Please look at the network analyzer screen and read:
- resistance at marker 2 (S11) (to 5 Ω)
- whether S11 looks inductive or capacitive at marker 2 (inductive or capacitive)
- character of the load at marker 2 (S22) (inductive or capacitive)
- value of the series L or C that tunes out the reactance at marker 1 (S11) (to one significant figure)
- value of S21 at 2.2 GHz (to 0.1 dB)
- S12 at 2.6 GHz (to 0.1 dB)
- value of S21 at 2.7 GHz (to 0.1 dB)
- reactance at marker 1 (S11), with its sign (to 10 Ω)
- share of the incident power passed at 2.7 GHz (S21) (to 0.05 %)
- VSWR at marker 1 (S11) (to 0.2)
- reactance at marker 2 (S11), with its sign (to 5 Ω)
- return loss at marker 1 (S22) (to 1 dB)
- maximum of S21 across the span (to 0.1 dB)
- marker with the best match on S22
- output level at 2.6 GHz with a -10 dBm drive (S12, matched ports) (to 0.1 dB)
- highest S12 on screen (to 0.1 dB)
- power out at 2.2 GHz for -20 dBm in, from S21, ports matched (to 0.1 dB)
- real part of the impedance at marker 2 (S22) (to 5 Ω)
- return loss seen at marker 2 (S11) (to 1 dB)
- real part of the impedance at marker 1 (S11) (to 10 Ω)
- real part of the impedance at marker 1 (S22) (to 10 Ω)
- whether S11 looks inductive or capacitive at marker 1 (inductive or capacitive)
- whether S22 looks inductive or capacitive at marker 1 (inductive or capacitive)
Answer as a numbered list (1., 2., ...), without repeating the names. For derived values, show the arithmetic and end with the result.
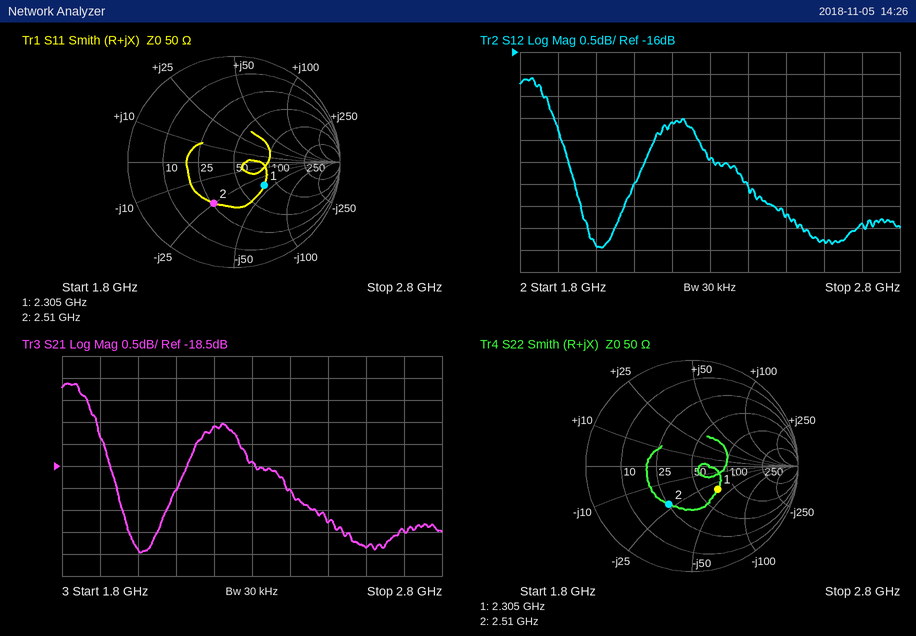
1. 25 Ω
2. capacitive
3. capacitive
4. L = 40 Ω/(2π × 2.305 GHz) ≈ 3 nH
5. -17.6 dB
6. -20.3 dB
7. -20.0 dB
8. -40 Ω
9. 10^(-20/10) ≈ 1.00 %
10. 2.2
11. -25 Ω
12. 10 dB
13. -16.6 dB
14. marker 1
15. -10 dBm + (-20.3 dB) = -30.3 dBm
16. -16.6 dB
17. -20 dBm + (-17.6 dB) = -37.6 dBm
18. 25 Ω
19. 7 dB
20. 80 Ω
21. 70 Ω
22. capacitive
23. capacitive
